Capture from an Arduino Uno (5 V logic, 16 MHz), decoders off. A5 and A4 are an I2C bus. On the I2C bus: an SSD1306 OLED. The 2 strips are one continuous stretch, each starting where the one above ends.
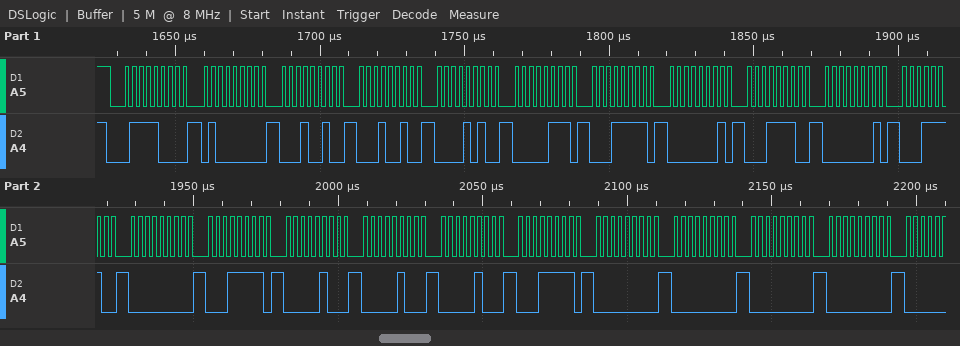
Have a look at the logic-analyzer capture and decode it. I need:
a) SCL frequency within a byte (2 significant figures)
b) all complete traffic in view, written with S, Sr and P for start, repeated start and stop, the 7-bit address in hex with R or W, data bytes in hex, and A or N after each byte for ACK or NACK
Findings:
400 kHz
S 3CW A 40 A 12 A 12 A 0A A 07 A 1F A 01 A 1E A 01 A 1E A 00 A 1F A 04 A 04 A 04 A 1F A 00 A 00 A 00 A 00 A
